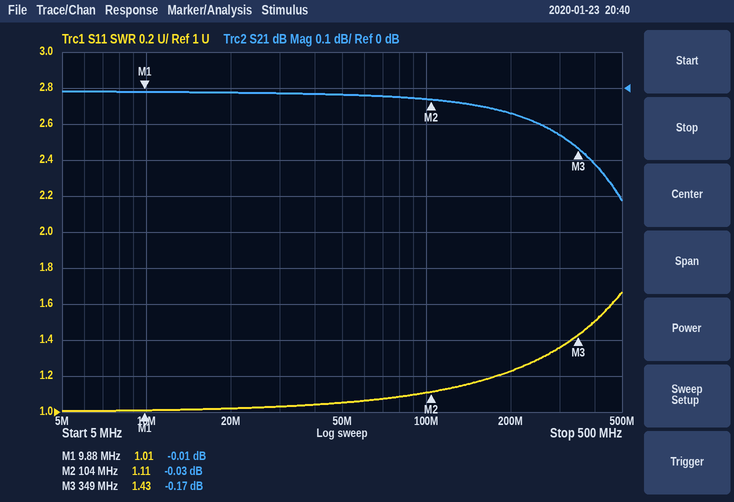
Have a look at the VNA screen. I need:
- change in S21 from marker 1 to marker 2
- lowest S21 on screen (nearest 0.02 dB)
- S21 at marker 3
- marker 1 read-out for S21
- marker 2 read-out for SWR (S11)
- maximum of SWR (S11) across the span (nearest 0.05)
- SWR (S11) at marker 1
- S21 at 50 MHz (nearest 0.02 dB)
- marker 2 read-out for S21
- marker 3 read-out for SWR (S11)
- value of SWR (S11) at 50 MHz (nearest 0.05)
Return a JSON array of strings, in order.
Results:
["-0.02 dB", "-0.32 dB", "-0.17 dB", "-0.01 dB", "1.11", "1.65", "1.01", "-0.02 dB", "-0.03 dB", "1.43", "1.05"]
